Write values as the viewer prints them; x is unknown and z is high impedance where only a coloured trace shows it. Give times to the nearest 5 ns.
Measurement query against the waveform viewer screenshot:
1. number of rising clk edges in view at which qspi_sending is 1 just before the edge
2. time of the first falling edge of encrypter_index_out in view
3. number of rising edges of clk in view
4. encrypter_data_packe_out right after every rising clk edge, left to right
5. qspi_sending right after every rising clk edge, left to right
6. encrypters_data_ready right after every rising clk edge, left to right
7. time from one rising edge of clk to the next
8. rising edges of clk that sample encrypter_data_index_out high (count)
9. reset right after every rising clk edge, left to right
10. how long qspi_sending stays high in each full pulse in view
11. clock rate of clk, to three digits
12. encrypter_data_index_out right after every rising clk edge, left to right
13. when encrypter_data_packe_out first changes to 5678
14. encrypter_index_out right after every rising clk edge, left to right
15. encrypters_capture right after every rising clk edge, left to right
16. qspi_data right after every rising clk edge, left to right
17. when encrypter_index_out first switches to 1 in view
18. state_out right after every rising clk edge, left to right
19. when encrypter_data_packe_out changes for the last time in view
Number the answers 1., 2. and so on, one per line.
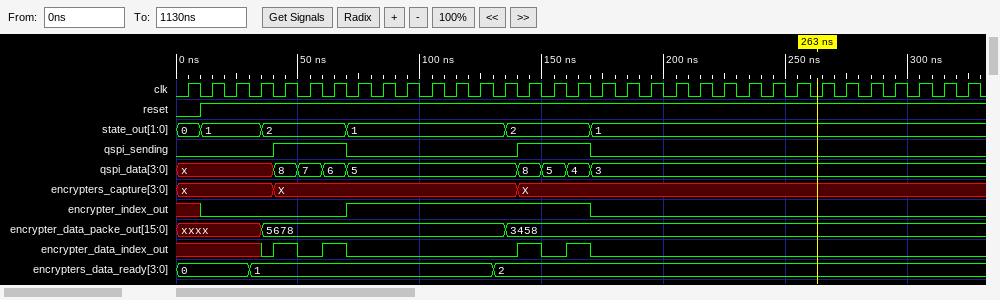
1. 6
2. 170 ns
3. 33
4. xxxx, xxxx, xxxx, 5678, 5678, 5678, 5678, 5678, 5678, 5678, 5678, 5678, 5678, 3458, 3458, 3458, 3458, 3458, 3458, 3458, 3458, 3458, 3458, 3458, 3458, 3458, 3458, 3458, 3458, 3458, 3458, 3458, 3458
5. 0 0 0 0 1 1 1 0 0 0 0 0 0 0 1 1 1 0 0 0 0 0 0 0 0 0 0 0 0 0 0 0 0
6. 0, 0, 0, 1, 1, 1, 1, 1, 1, 1, 1, 1, 1, 2, 2, 2, 2, 2, 2, 2, 2, 2, 2, 2, 2, 2, 2, 2, 2, 2, 2, 2, 2
7. 10 ns
8. 4
9. 0 1 1 1 1 1 1 1 1 1 1 1 1 1 1 1 1 1 1 1 1 1 1 1 1 1 1 1 1 1 1 1 1
10. 30 ns, 30 ns
11. 100 MHz
12. x x x 0 1 0 1 0 0 0 0 0 0 0 1 0 1 0 0 0 0 0 0 0 0 0 0 0 0 0 0 0 0
13. 35 ns
14. x 0 0 0 0 0 0 1 1 1 1 1 1 1 1 1 1 0 0 0 0 0 0 0 0 0 0 0 0 0 0 0 0
15. x, x, x, x, X, X, X, X, X, X, X, X, X, X, X, X, X, X, X, X, X, X, X, X, X, X, X, X, X, X, X, X, X
16. x, x, x, x, 8, 7, 6, 5, 5, 5, 5, 5, 5, 5, 8, 5, 4, 3, 3, 3, 3, 3, 3, 3, 3, 3, 3, 3, 3, 3, 3, 3, 3
17. 70 ns
18. 0, 1, 1, 2, 2, 2, 2, 1, 1, 1, 1, 1, 1, 2, 2, 2, 2, 1, 1, 1, 1, 1, 1, 1, 1, 1, 1, 1, 1, 1, 1, 1, 1
19. 135 ns
